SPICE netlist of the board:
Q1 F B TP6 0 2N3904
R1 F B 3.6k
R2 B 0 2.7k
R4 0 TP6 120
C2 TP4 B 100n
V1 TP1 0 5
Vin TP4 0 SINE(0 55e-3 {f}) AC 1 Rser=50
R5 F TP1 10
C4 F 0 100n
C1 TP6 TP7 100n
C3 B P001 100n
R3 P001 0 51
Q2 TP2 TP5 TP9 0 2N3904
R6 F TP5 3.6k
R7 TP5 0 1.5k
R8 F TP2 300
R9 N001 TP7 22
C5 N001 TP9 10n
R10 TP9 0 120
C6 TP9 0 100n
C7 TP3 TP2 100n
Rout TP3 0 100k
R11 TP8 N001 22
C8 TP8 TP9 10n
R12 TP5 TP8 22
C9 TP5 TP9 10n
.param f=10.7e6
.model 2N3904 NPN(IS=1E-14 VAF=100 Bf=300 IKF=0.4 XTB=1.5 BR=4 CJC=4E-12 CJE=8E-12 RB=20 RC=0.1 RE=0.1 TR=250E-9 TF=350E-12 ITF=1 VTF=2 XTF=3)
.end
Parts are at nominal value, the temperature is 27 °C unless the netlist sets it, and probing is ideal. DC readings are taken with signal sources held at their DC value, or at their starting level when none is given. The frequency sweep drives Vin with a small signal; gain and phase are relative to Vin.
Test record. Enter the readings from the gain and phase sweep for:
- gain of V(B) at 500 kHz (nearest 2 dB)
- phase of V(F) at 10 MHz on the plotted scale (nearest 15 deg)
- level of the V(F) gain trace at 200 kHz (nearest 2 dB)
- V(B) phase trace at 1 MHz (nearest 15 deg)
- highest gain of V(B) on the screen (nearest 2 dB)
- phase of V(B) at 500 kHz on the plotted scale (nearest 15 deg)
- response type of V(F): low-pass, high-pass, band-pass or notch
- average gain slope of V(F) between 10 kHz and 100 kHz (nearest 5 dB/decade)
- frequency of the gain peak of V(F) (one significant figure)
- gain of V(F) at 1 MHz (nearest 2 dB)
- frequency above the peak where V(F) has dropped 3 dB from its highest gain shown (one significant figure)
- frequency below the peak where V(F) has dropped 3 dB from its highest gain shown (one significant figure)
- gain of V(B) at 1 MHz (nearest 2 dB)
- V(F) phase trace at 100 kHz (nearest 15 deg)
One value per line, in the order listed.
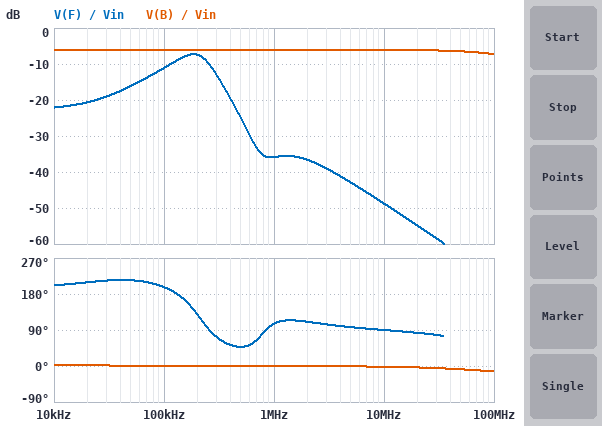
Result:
-6 dB
90 deg
-8 dB
0 deg
-6 dB
0 deg
band-pass
10 dB/decade
200 kHz
-36 dB
300 kHz
100 kHz
-6 dB
195 deg
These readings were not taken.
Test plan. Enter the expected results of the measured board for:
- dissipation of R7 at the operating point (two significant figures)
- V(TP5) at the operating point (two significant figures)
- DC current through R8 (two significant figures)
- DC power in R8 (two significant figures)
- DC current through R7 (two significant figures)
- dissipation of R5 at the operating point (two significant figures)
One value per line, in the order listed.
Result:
1.3 mW
1.4 V
5.8 mA
10 mW
930 µA
3.3 mW
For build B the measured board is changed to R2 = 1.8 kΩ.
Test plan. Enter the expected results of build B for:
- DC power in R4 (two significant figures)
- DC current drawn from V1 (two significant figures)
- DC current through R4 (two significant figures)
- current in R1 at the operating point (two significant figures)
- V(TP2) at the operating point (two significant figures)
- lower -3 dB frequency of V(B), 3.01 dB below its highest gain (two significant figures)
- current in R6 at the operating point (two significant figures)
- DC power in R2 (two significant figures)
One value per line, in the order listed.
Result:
6.5 mW
15 mA
7.3 mA
910 µA
3.1 V
710 Hz
960 µA
1.4 mW
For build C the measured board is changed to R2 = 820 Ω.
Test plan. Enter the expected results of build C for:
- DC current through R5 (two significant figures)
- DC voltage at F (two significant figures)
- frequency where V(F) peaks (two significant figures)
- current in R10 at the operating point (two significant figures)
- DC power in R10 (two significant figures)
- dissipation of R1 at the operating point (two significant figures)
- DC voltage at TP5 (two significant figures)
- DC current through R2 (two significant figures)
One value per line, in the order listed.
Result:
10 mA
4.9 V
180 kHz
6.0 mA
4.3 mW
4.4 mW
1.4 V
1.1 mA
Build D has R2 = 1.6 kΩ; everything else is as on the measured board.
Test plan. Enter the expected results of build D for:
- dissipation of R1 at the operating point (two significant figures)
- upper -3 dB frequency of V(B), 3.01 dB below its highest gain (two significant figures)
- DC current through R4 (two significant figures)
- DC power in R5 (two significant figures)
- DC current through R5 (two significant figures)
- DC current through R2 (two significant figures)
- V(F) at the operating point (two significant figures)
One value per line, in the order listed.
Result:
3.2 mW
250 MHz
6.4 mA
2.0 mW
14 mA
920 µA
4.9 V
